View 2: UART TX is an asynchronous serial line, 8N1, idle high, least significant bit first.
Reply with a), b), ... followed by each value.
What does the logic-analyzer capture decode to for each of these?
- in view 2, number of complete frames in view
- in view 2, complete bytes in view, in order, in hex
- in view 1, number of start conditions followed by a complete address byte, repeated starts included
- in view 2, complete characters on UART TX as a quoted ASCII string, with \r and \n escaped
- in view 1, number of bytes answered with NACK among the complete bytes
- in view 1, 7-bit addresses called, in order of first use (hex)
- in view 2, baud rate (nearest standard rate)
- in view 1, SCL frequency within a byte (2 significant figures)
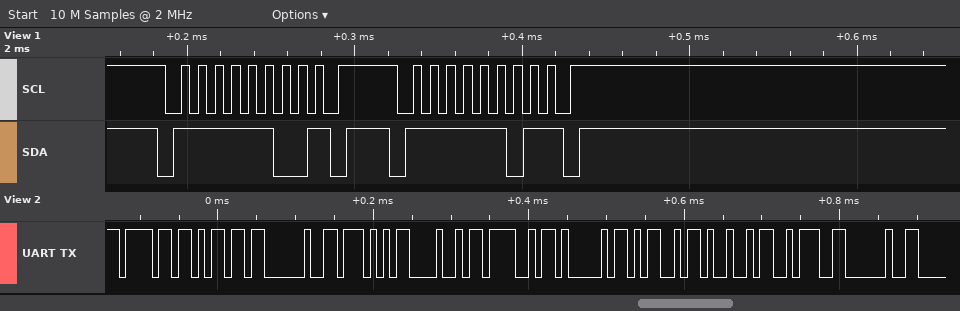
a) 11
b) 6F 6D 20 57 48 4F 41 4D 49 3A 20
c) 2
d) "om WHOAMI: "
e) 2
f) 0x7E
g) 115200 baud
h) 100 kHz
